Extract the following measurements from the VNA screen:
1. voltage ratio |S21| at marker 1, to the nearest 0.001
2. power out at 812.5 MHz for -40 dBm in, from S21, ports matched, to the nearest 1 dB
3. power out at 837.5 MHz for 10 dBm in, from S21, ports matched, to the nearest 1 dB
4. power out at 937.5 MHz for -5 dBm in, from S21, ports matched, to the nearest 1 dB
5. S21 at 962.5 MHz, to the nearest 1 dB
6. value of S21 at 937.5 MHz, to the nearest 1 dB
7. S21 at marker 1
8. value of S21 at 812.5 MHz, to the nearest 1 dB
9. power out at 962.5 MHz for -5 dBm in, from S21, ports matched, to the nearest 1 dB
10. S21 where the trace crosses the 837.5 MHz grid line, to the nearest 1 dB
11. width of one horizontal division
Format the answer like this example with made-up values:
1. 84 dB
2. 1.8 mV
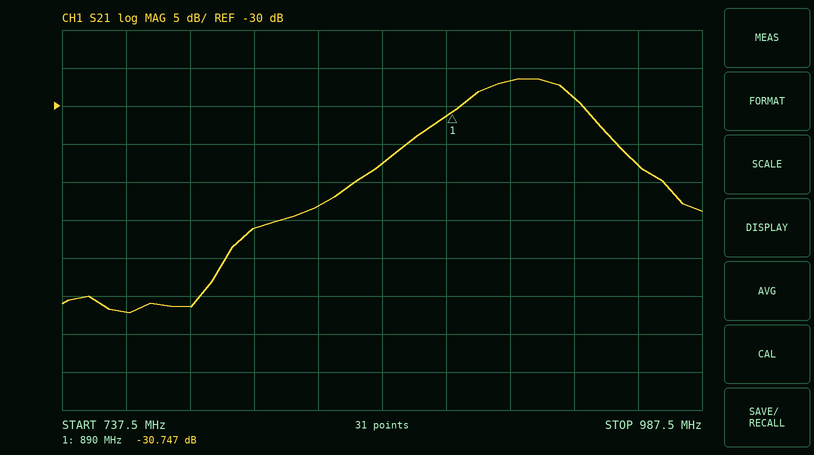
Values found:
1. 0.029
2. -86 dBm
3. -33 dBm
4. -34 dBm
5. -38 dB
6. -29 dB
7. -30.747 dB
8. -46 dB
9. -43 dBm
10. -43 dB
11. 25 MHz
